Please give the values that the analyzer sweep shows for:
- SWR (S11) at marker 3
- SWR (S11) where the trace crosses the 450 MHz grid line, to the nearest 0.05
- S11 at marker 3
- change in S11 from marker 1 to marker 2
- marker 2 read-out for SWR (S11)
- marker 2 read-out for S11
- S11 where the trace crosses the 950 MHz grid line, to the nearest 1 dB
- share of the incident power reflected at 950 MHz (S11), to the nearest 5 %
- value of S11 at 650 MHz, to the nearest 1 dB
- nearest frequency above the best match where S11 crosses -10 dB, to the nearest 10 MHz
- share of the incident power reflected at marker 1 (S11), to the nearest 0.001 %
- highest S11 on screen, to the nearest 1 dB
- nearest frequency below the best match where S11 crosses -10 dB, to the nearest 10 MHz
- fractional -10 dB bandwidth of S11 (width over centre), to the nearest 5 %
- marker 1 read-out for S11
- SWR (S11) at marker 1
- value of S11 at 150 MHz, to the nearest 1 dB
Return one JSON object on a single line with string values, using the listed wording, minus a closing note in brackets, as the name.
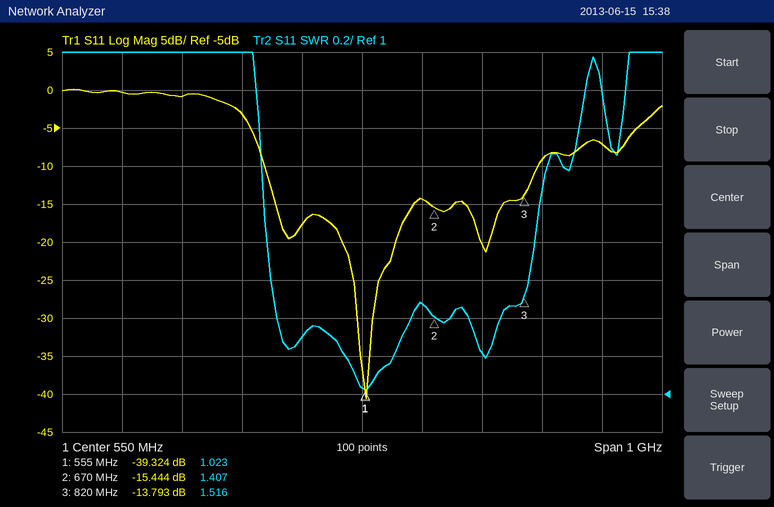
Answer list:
{"SWR (S11) at marker 3": "1.516", "SWR (S11) where the trace crosses the 450 MHz grid line, to the nearest 0.05": "1.30", "S11 at marker 3": "-13.793 dB", "change in S11 from marker 1 to marker 2": "23.880 dB", "marker 2 read-out for SWR": "1.407", "marker 2 read-out for S11": "-15.444 dB", "S11 where the trace crosses the 950 MHz grid line, to the nearest 1 dB": "-7 dB", "share of the incident power reflected at 950 MHz (S11), to the nearest 5 %": "20 %", "value of S11 at 650 MHz, to the nearest 1 dB": "-14 dB", "nearest frequency above the best match where S11 crosses -10 dB, to the nearest 10 MHz": "840 MHz", "share of the incident power reflected at marker 1 (S11), to the nearest 0.001 %": "0.012 %", "highest S11 on screen, to the nearest 1 dB": "0 dB", "nearest frequency below the best match where S11 crosses -10 dB, to the nearest 10 MHz": "390 MHz", "fractional -10 dB bandwidth of S11 (width over centre), to the nearest 5 %": "75 %", "marker 1 read-out for S11": "-39.324 dB", "SWR (S11) at marker 1": "1.023", "value of S11 at 150 MHz, to the nearest 1 dB": "0 dB"}
